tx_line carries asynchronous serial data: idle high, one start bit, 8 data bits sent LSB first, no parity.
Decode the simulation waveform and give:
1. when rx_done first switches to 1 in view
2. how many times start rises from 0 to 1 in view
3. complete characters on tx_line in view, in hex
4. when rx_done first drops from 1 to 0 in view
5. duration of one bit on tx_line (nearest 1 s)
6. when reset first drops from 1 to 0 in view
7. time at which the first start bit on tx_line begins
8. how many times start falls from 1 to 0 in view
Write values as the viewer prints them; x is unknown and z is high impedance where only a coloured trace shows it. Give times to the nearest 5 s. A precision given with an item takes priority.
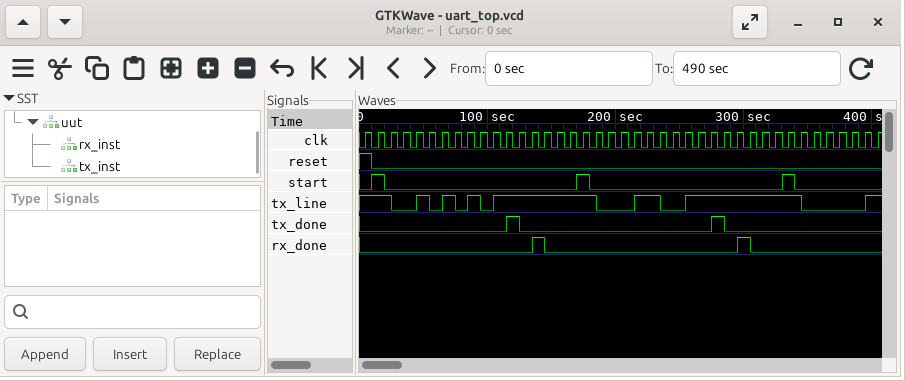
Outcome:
135 s
3
AA, CC
145 s
10 s
10 s
25 s
3
